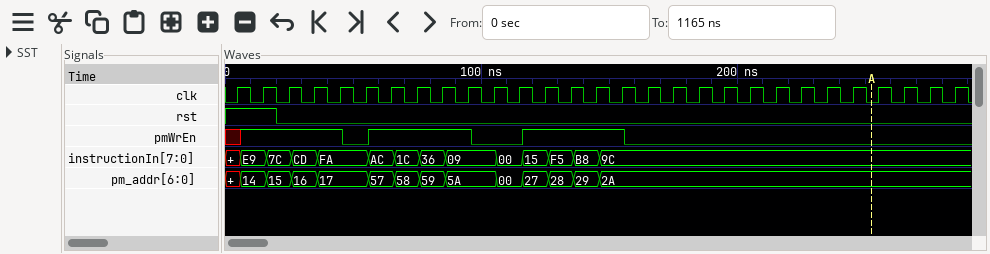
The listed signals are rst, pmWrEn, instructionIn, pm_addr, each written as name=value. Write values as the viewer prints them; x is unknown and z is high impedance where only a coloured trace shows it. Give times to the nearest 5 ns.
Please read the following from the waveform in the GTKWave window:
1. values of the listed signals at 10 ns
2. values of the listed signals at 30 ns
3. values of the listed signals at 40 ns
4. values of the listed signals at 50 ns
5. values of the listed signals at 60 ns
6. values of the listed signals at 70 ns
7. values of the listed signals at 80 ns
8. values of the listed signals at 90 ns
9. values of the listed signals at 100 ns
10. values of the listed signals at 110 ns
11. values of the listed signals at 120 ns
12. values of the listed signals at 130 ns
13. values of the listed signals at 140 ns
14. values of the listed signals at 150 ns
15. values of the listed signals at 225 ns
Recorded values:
rst=1, pmWrEn=1, instructionIn=E9, pm_addr=14
rst=0, pmWrEn=1, instructionIn=CD, pm_addr=16
rst=0, pmWrEn=1, instructionIn=FA, pm_addr=17
rst=0, pmWrEn=0, instructionIn=FA, pm_addr=17
rst=0, pmWrEn=1, instructionIn=AC, pm_addr=57
rst=0, pmWrEn=1, instructionIn=1C, pm_addr=58
rst=0, pmWrEn=1, instructionIn=36, pm_addr=59
rst=0, pmWrEn=1, instructionIn=09, pm_addr=5A
rst=0, pmWrEn=0, instructionIn=09, pm_addr=5A
rst=0, pmWrEn=0, instructionIn=00, pm_addr=00
rst=0, pmWrEn=1, instructionIn=15, pm_addr=27
rst=0, pmWrEn=1, instructionIn=F5, pm_addr=28
rst=0, pmWrEn=1, instructionIn=B8, pm_addr=29
rst=0, pmWrEn=1, instructionIn=9C, pm_addr=2A
rst=0, pmWrEn=0, instructionIn=9C, pm_addr=2A
